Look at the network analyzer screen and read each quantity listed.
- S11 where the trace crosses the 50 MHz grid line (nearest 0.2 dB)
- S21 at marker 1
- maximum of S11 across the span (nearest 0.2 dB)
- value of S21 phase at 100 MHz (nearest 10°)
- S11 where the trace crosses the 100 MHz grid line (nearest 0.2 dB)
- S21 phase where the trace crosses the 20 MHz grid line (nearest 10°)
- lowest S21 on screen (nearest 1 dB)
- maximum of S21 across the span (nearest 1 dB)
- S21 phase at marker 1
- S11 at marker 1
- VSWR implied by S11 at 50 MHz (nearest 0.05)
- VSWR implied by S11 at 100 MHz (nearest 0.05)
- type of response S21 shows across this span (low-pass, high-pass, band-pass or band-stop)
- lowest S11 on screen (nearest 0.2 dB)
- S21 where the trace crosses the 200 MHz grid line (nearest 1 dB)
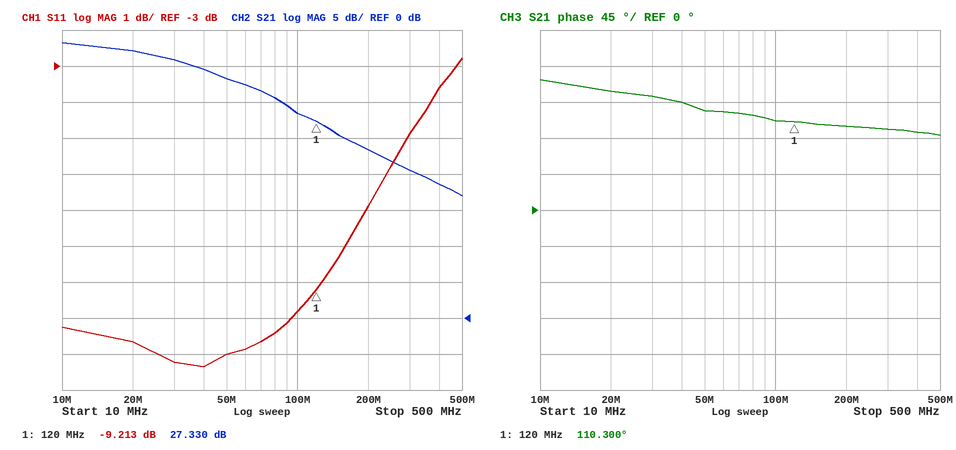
-11.0 dB
27.330 dB
-2.8 dB
110°
-9.8 dB
150°
17 dB
38 dB
110.300°
-9.213 dB
1.80
1.95
low-pass
-11.4 dB
23 dB
